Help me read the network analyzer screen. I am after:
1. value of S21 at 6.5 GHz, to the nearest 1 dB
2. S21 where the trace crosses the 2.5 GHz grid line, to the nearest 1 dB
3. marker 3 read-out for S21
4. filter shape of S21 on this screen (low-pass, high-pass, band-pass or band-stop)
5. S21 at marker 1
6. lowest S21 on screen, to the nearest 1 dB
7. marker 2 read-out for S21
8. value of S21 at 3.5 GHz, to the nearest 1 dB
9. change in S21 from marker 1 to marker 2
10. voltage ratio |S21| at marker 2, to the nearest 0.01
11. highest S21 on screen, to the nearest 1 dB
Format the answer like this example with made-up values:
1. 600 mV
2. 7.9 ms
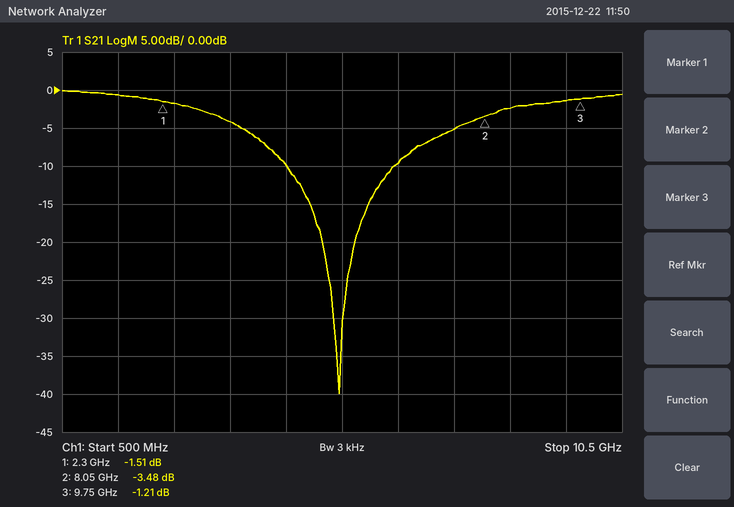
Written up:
1. -10 dB
2. -2 dB
3. -1.21 dB
4. band-stop
5. -1.51 dB
6. -40 dB
7. -3.48 dB
8. -4 dB
9. -1.97 dB
10. 0.67
11. 0 dB
